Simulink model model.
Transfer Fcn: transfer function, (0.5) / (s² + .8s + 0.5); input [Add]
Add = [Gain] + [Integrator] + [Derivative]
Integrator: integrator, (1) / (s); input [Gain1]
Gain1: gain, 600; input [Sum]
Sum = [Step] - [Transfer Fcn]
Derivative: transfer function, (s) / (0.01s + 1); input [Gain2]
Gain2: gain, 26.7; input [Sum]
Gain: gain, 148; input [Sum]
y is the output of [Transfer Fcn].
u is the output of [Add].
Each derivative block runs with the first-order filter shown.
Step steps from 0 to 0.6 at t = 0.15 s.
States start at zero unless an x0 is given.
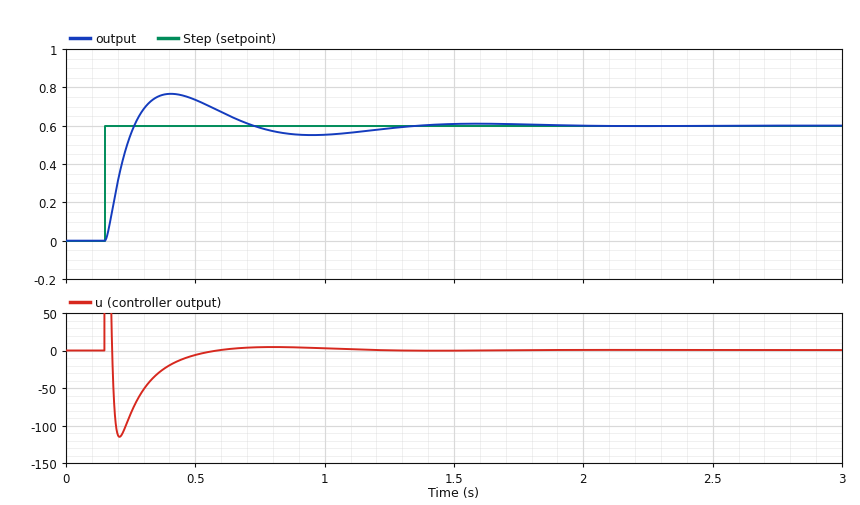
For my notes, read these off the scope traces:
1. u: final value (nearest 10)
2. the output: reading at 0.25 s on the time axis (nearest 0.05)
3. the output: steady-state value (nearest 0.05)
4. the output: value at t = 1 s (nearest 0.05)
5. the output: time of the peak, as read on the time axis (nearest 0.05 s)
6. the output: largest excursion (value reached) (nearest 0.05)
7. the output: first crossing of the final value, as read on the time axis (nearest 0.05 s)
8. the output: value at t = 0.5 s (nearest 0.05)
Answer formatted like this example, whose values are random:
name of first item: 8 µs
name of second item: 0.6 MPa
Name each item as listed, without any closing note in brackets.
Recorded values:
u: final value: 0
the output: reading at 0.25 s on the time axis: 0.55
the output: steady-state value: 0.60
the output: value at t = 1 s: 0.55
the output: time of the peak, as read on the time axis: 0.40 s
the output: largest excursion (value reached): 0.75
the output: first crossing of the final value, as read on the time axis: 0.25 s
the output: value at t = 0.5 s: 0.75
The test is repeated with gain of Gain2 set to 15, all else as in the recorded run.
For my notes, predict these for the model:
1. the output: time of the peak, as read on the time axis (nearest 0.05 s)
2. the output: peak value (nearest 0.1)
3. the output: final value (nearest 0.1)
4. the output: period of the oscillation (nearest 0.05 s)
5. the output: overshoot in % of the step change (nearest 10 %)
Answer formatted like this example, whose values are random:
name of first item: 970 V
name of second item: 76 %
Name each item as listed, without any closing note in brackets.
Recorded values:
the output: time of the peak, as read on the time axis: 0.45 s
the output: peak value: 0.9
the output: final value: 0.6
the output: period of the oscillation: 0.80 s
the output: overshoot in % of the step change: 50 %
